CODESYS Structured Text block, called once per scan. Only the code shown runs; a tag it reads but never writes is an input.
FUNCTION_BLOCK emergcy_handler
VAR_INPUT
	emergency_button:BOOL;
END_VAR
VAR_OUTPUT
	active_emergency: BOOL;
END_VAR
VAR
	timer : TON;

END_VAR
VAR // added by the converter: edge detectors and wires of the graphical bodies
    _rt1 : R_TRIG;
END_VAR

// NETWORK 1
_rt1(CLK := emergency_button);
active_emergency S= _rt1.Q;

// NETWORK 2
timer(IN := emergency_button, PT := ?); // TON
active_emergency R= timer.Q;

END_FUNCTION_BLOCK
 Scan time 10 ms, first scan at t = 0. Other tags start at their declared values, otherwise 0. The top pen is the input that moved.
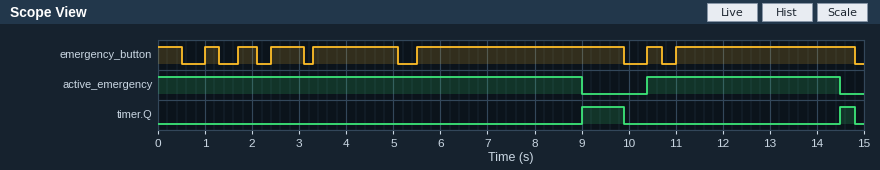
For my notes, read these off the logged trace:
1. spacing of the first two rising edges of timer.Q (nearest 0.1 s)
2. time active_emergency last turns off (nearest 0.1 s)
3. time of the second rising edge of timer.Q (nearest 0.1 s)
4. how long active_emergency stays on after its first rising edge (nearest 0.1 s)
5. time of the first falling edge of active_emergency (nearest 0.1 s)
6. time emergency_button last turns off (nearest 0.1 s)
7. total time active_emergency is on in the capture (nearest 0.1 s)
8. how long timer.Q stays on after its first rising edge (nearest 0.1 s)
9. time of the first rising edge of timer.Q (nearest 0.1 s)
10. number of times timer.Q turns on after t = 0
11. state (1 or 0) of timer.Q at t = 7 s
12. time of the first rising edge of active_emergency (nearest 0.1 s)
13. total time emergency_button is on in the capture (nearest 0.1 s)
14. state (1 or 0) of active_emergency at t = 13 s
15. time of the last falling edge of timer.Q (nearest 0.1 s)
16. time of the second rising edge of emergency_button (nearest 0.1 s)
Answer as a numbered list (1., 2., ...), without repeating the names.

1. 5.5 s
2. 14.5 s
3. 14.5 s
4. 4.1 s
5. 9.0 s
6. 14.8 s
7. 13.1 s
8. 0.9 s
9. 9.0 s
10. 2
11. 0
12. 10.4 s
13. 12.2 s
14. 1
15. 14.8 s
16. 1.7 s
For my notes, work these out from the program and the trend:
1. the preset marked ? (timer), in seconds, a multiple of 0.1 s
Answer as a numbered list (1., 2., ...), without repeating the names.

1. 3.5 s
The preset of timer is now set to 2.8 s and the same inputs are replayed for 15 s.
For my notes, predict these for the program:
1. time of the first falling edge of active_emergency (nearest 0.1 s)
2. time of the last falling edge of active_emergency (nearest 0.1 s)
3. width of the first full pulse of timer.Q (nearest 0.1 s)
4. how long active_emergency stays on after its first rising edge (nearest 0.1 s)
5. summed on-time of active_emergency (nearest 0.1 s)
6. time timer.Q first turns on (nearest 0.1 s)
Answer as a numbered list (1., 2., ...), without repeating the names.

1. 8.3 s
2. 13.8 s
3. 1.6 s
4. 3.4 s
5. 11.7 s
6. 8.3 s
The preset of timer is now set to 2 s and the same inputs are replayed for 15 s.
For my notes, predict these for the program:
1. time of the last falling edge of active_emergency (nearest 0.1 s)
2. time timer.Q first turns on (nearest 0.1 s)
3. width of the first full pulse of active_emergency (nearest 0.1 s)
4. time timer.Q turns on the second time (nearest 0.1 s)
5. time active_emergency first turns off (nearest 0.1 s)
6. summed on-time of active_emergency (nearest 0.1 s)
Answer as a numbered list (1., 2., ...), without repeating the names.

1. 13.0 s
2. 7.5 s
3. 2.6 s
4. 13.0 s
5. 7.5 s
6. 10.1 s
